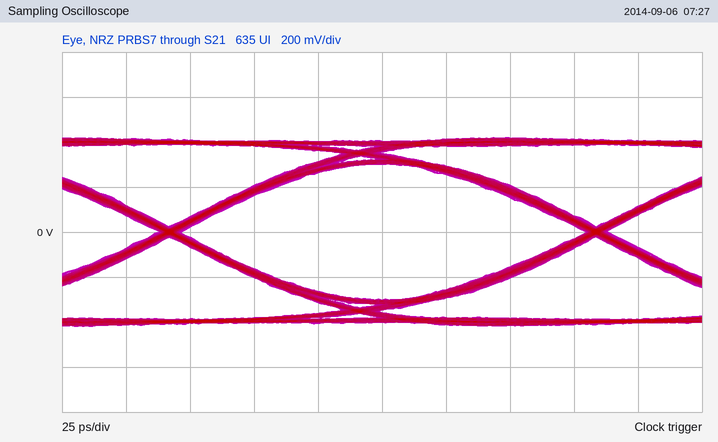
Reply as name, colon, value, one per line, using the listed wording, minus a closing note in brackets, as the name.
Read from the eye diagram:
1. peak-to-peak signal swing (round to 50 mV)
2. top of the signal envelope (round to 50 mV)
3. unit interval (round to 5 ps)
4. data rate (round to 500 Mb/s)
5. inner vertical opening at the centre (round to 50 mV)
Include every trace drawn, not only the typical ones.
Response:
peak-to-peak signal swing: 850 mV
top of the signal envelope: 400 mV
unit interval: 165 ps
data rate: 6.0 Gb/s
inner vertical opening at the centre: 600 mV
